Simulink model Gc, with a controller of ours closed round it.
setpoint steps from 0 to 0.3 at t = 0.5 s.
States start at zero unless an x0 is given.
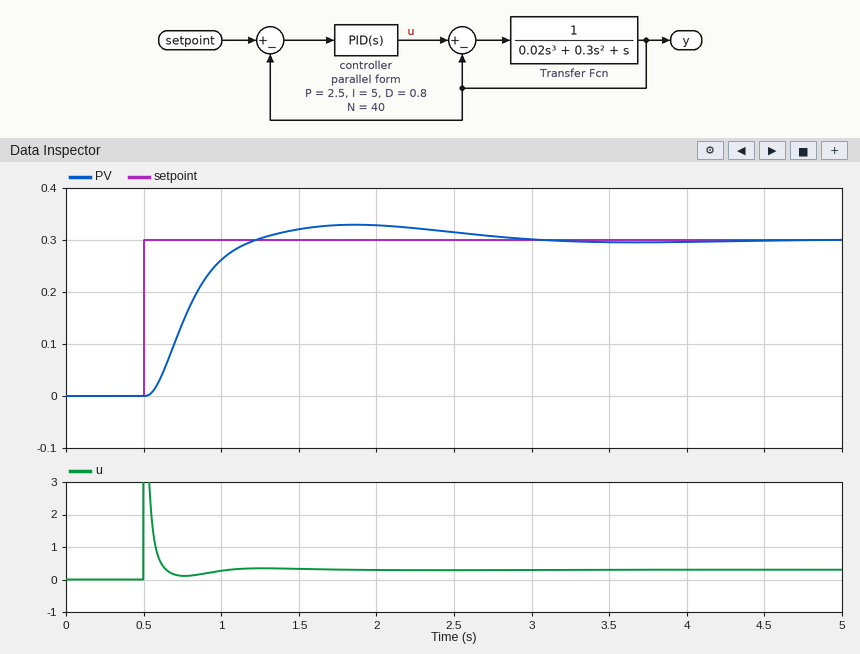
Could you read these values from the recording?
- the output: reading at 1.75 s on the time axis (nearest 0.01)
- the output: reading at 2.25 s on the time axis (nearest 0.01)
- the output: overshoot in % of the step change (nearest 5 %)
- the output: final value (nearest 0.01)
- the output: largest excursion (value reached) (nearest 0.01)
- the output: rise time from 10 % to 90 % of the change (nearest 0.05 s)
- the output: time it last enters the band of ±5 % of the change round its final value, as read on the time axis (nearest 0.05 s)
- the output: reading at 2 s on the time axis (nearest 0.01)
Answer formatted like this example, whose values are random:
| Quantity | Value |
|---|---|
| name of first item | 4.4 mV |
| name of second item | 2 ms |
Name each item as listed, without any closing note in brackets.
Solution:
| Quantity | Value |
|---|---|
| the output: reading at 1.75 s on the time axis | 0.33 |
| the output: reading at 2.25 s on the time axis | 0.32 |
| the output: overshoot in % of the step change | 10 % |
| the output: final value | 0.30 |
| the output: largest excursion (value reached) | 0.33 |
| the output: rise time from 10 % to 90 % of the change | 0.45 s |
| the output: time it last enters the band of ±5 % of the change round its final value, as read on the time axis | 2.50 s |
| the output: reading at 2 s on the time axis | 0.33 |
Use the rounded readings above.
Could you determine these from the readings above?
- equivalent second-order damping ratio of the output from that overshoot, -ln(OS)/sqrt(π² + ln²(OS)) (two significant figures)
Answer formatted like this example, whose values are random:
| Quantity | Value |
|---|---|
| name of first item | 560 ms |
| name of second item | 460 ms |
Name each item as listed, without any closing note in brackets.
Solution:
| Quantity | Value |
|---|---|
| equivalent second-order damping ratio of the output from that overshoot, -ln(OS)/sqrt(π² + ln²(OS)) | 0.59 |
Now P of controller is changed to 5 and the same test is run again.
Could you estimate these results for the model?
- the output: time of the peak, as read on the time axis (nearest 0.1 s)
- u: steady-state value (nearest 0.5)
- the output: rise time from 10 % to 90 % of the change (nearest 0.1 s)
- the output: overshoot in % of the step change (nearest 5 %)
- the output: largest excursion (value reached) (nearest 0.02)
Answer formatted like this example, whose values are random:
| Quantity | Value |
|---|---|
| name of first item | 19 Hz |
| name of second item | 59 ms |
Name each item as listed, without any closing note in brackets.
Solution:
| Quantity | Value |
|---|---|
| the output: time of the peak, as read on the time axis | 1.1 s |
| u: steady-state value | 0.5 |
| the output: rise time from 10 % to 90 % of the change | 0.3 s |
| the output: overshoot in % of the step change | 15 % |
| the output: largest excursion (value reached) | 0.34 |
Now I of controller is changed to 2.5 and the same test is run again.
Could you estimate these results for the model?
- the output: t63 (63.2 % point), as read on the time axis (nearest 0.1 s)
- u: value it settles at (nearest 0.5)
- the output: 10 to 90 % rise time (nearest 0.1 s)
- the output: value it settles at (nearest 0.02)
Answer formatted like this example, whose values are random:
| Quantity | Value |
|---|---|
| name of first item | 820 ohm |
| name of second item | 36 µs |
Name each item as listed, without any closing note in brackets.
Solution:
| Quantity | Value |
|---|---|
| the output: t63 (63.2 % point), as read on the time axis | 0.8 s |
| u: value it settles at | 0.5 |
| the output: 10 to 90 % rise time | 0.8 s |
| the output: value it settles at | 0.30 |
